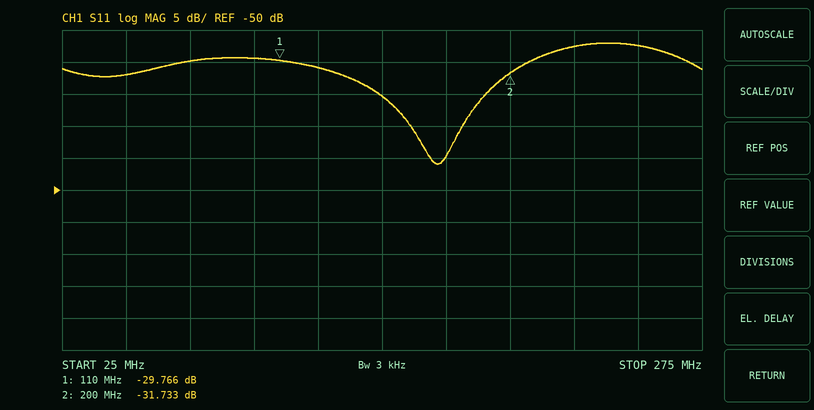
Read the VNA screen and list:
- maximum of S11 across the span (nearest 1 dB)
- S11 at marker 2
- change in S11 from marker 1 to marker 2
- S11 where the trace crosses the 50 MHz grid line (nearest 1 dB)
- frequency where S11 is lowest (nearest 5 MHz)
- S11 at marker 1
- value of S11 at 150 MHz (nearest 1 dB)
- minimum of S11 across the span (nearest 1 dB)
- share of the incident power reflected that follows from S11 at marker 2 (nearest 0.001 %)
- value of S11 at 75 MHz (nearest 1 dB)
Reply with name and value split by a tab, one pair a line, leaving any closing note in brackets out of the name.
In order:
maximum of S11 across the span	-27 dB
S11 at marker 2	-31.733 dB
change in S11 from marker 1 to marker 2	-1.967 dB
S11 where the trace crosses the 50 MHz grid line	-32 dB
frequency where S11 is lowest	170 MHz
S11 at marker 1	-29.766 dB
value of S11 at 150 MHz	-35 dB
minimum of S11 across the span	-46 dB
share of the incident power reflected that follows from S11 at marker 2	0.067 %
value of S11 at 75 MHz	-30 dB
